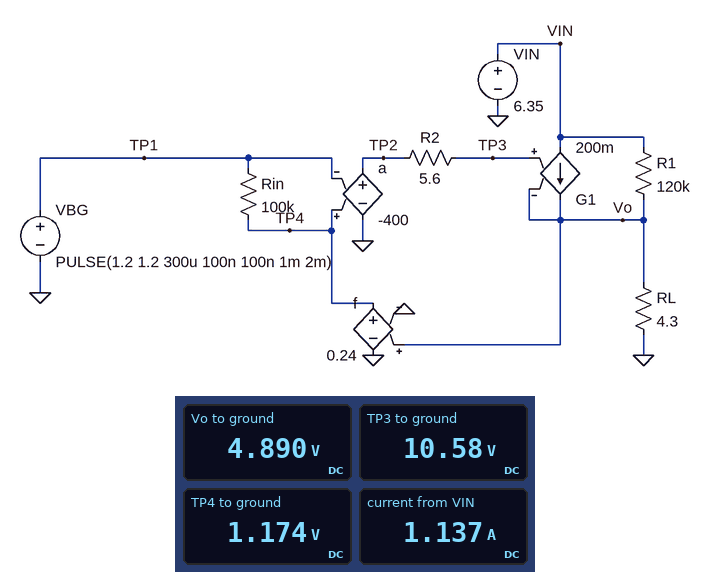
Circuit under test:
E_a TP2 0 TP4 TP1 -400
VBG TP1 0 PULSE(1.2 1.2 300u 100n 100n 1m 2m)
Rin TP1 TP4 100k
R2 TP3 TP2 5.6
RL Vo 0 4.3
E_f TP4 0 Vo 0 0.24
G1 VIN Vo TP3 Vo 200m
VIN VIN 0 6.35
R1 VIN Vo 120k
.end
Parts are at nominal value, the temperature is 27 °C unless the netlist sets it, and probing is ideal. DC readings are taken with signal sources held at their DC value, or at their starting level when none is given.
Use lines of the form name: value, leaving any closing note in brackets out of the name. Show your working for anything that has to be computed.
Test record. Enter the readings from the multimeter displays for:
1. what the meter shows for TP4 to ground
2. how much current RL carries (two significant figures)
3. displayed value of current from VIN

what the meter shows for TP4 to ground: 1.174 V
how much current RL carries: (4.89 V) / 4.3 Ω = 1.1 A
displayed value of current from VIN: 1.137 A
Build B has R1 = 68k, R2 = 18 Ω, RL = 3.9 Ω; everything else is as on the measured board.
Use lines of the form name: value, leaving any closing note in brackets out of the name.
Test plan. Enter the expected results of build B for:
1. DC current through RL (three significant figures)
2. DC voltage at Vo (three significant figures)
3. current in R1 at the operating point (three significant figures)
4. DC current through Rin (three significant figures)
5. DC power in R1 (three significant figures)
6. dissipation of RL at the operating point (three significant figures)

DC current through RL: 1.25 A
DC voltage at Vo: 4.88 V
current in R1 at the operating point: 21.6 µA
DC current through Rin: 279 nA
DC power in R1: 31.6 µW
dissipation of RL at the operating point: 6.12 W
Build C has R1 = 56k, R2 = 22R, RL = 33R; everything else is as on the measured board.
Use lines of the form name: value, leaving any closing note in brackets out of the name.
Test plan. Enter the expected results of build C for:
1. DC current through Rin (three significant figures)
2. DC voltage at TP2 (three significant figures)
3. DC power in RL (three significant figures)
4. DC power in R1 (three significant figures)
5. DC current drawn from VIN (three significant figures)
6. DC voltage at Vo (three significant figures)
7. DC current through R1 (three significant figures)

DC current through Rin: 142 nA
DC voltage at TP2: 5.69 V
DC power in RL: 740 mW
DC power in R1: 35.5 µW
DC current drawn from VIN: 150 mA
DC voltage at Vo: 4.94 V
DC current through R1: 25.2 µA
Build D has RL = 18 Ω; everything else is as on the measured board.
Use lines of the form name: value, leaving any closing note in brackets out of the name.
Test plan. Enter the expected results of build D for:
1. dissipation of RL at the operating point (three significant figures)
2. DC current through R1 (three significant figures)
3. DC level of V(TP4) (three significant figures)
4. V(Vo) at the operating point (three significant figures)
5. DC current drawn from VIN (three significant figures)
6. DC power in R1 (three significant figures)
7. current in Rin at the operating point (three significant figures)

dissipation of RL at the operating point: 1.35 W
DC current through R1: 11.8 µA
DC level of V(TP4): 1.18 V
V(Vo) at the operating point: 4.93 V
DC current drawn from VIN: 274 mA
DC power in R1: 16.7 µW
current in Rin at the operating point: 158 nA
